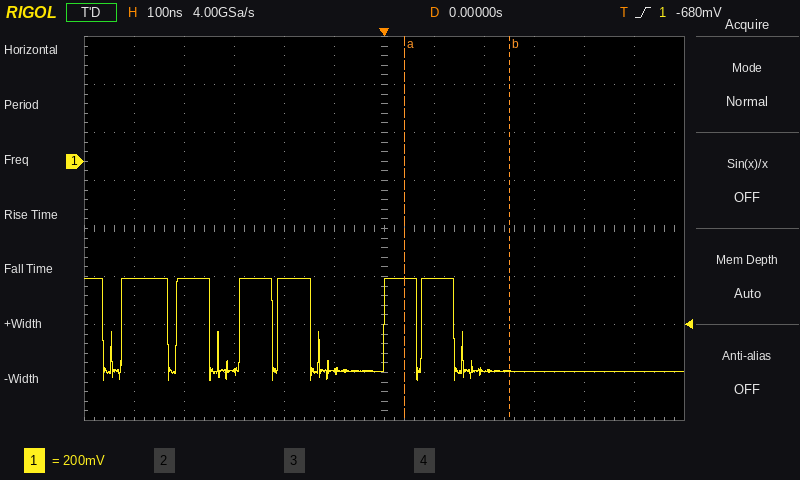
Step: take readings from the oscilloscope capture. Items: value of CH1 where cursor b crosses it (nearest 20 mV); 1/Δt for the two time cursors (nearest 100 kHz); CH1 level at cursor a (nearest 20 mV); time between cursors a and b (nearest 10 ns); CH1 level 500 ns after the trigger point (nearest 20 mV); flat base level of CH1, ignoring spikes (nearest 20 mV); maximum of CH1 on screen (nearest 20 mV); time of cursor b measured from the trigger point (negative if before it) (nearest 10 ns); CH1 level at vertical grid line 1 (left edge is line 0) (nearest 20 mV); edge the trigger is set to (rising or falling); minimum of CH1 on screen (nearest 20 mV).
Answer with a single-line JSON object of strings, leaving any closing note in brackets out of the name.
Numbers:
{"value of CH1 where cursor b crosses it": "-880 mV", "1/Δt for the two time cursors": "4.8 MHz", "CH1 level at cursor a": "-480 mV", "time between cursors a and b": "210 ns", "CH1 level 500 ns after the trigger point": "-880 mV", "flat base level of CH1, ignoring spikes": "-880 mV", "maximum of CH1 on screen": "-480 mV", "time of cursor b measured from the trigger point (negative if before it)": "+250 ns", "CH1 level at vertical grid line 1 (left edge is line 0)": "-480 mV", "edge the trigger is set to": "rising", "minimum of CH1 on screen": "-920 mV"}
